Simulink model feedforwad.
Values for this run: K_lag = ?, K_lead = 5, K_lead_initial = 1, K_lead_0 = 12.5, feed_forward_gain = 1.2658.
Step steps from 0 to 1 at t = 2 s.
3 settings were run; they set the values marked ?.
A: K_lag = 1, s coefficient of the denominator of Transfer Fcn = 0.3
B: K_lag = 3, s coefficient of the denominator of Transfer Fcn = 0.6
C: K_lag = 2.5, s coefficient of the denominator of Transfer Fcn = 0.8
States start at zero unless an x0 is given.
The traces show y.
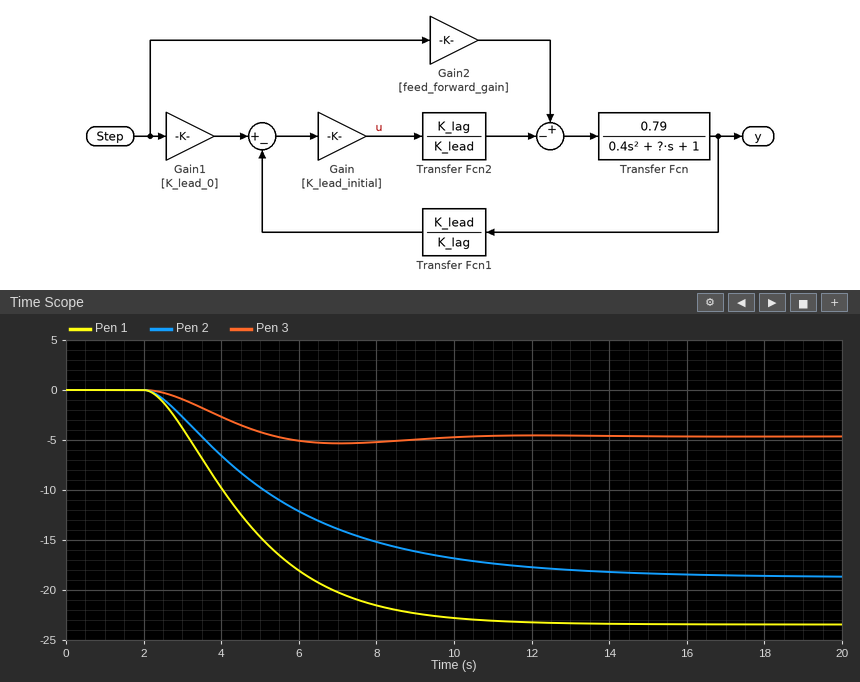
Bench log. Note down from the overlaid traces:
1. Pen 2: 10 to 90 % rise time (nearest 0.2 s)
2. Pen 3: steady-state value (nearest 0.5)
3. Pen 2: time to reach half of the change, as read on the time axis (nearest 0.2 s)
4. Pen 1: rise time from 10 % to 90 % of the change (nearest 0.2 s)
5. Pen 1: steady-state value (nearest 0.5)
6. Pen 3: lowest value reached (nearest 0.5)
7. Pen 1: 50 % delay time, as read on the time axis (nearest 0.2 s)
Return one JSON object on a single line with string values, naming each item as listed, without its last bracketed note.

{"Pen 2: 10 to 90 % rise time": "7.2 s", "Pen 3: steady-state value": "-4.5", "Pen 2: time to reach half of the change, as read on the time axis": "4.8 s", "Pen 1: rise time from 10 % to 90 % of the change": "4.8 s", "Pen 1: steady-state value": "-23.5", "Pen 3: lowest value reached": "-5.5", "Pen 1: 50 % delay time, as read on the time axis": "4.4 s"}
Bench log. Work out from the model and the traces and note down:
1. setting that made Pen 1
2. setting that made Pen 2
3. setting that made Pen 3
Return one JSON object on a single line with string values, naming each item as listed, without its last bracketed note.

{"setting that made Pen 1": "B", "setting that made Pen 2": "C", "setting that made Pen 3": "A"}
